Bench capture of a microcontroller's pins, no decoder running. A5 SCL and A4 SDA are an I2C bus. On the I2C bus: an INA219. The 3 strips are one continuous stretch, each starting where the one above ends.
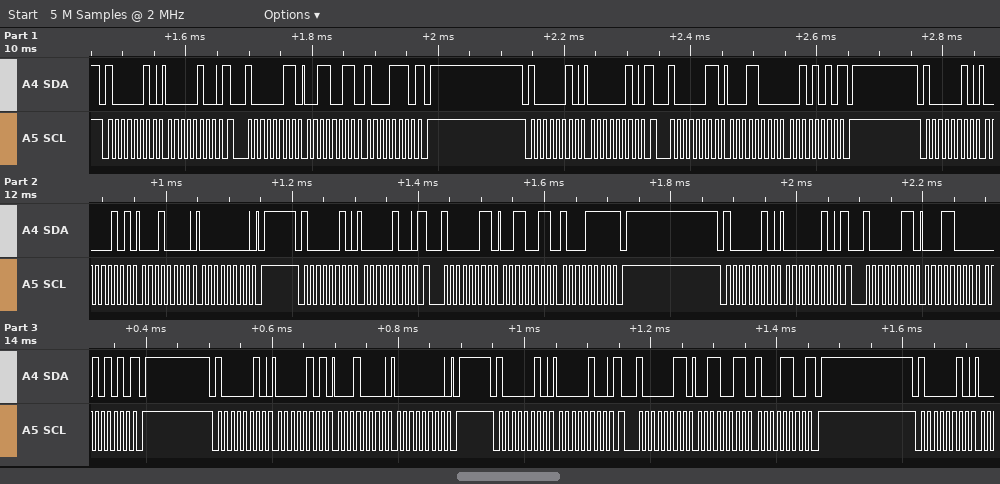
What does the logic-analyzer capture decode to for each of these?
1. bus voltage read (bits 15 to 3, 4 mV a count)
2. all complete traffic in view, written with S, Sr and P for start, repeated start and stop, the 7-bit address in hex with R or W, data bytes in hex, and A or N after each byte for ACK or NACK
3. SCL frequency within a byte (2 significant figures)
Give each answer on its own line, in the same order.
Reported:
3.092 V
S 41W A 04 A Sr 41R A 33 A 8E N P S 41W A 02 A Sr 41R A 18 A 2A N P S 41W A 05 A 10 A 00 A P S 41W A 04 A Sr 41R A 33 A 8F N P S 41W A 02 A Sr 41R A 18 A 2A N P S 41W A 05 A 10 A 00 A P S 41W A 04 A Sr 41R A 33 A 8C N P S 41W A
100 kHz
